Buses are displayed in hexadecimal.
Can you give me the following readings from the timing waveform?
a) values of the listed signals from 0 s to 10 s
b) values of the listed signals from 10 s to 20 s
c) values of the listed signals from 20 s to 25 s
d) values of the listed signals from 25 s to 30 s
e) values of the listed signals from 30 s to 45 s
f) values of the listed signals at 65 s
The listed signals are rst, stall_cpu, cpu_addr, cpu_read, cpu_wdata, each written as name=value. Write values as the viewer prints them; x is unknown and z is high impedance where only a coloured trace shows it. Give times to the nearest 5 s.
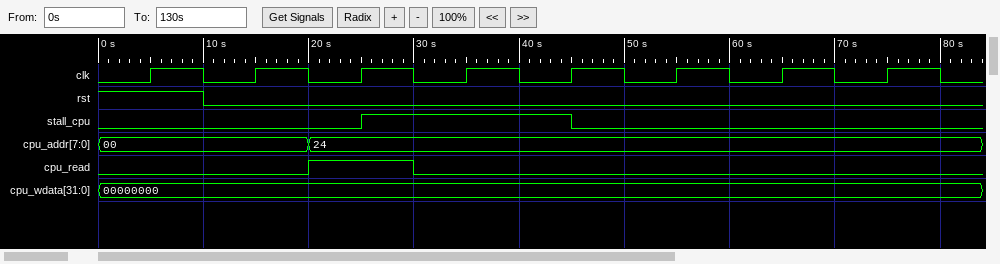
rst=1, stall_cpu=0, cpu_addr=00, cpu_read=0, cpu_wdata=00000000
rst=0, stall_cpu=0, cpu_addr=00, cpu_read=0, cpu_wdata=00000000
rst=0, stall_cpu=0, cpu_addr=24, cpu_read=1, cpu_wdata=00000000
rst=0, stall_cpu=1, cpu_addr=24, cpu_read=1, cpu_wdata=00000000
rst=0, stall_cpu=1, cpu_addr=24, cpu_read=0, cpu_wdata=00000000
rst=0, stall_cpu=0, cpu_addr=24, cpu_read=0, cpu_wdata=00000000
